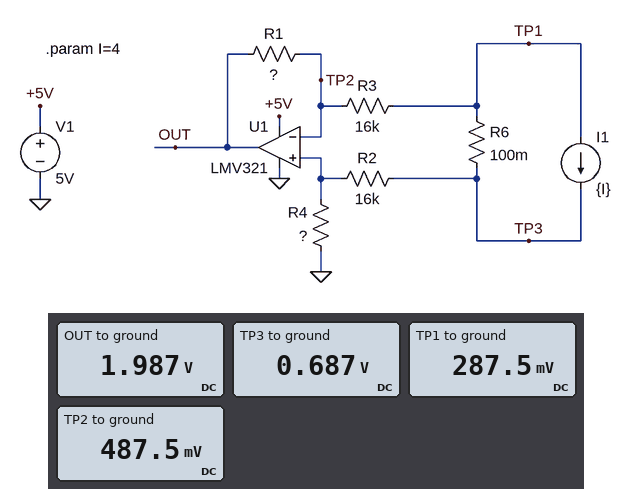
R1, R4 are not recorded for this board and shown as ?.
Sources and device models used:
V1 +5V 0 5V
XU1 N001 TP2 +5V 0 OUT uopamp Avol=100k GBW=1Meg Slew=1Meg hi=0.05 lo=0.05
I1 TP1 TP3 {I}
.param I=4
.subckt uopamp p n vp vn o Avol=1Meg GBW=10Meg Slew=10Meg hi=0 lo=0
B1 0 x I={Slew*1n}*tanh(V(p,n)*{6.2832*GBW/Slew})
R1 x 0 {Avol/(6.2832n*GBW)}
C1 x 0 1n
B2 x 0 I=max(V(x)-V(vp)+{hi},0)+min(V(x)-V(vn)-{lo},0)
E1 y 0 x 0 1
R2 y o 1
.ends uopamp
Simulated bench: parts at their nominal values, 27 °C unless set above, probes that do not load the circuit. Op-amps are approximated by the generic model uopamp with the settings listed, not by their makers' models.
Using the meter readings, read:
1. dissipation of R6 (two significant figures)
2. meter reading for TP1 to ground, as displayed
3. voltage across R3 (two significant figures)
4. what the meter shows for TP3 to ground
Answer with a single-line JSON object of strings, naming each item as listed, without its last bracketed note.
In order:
{"dissipation of R6": "1.6 W", "meter reading for TP1 to ground, as displayed": "287.5 mV", "voltage across R3": "200 mV", "what the meter shows for TP3 to ground": "0.687 V"}
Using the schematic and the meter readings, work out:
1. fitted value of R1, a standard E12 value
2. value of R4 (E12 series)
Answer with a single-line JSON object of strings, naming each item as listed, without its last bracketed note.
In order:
{"fitted value of R1, a standard E12 value": "120 kΩ", "value of R4": "39 kΩ"}
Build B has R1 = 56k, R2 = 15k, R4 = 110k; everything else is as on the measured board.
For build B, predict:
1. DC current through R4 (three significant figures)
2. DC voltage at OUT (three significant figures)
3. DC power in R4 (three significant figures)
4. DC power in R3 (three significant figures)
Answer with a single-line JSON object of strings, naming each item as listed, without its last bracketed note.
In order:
{"DC current through R4": "12.9 µA", "DC voltage at OUT": "2.14 V", "DC power in R4": "18.3 µW", "DC power in R3": "2.66 µW"}
